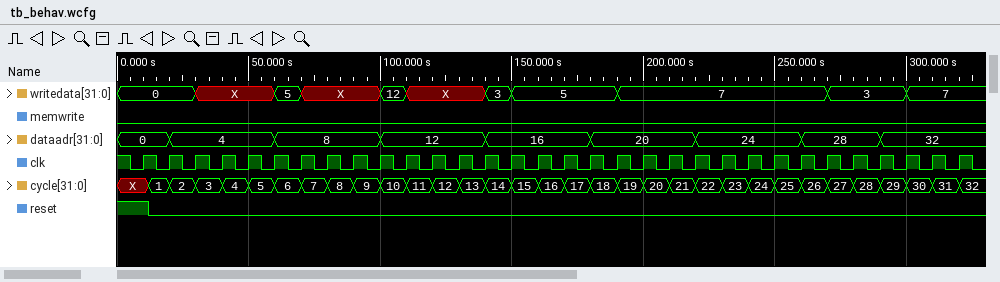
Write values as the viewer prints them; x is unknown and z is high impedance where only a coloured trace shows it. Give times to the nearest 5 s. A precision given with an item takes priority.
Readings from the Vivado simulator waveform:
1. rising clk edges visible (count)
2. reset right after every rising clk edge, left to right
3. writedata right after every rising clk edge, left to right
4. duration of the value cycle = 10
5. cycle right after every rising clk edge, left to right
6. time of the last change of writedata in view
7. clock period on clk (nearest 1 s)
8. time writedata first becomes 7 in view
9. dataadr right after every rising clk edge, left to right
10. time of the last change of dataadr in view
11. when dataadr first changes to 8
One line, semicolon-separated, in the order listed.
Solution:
32; 1 0 0 0 0 0 0 0 0 0 0 0 0 0 0 0 0 0 0 0 0 0 0 0 0 0 0 0 0 0 0 0; 0, 0, X, X, X, 5, X, X, X, 12, X, X, X, 3, 5, 5, 5, 5, 7, 7, 7, 7, 7, 7, 7, 7, 3, 3, 3, 7, 7, 7; 10 s; X, 2, 3, 4, 5, 6, 7, 8, 9, 10, 11, 12, 13, 14, 15, 16, 17, 18, 19, 20, 21, 22, 23, 24, 25, 26, 27, 28, 29, 30, 31, 32; 300 s; 10 s; 190 s; 0, 4, 4, 4, 4, 8, 8, 8, 8, 12, 12, 12, 12, 16, 16, 16, 16, 20, 20, 20, 20, 24, 24, 24, 24, 28, 28, 28, 32, 32, 32, 32; 290 s; 60 s
